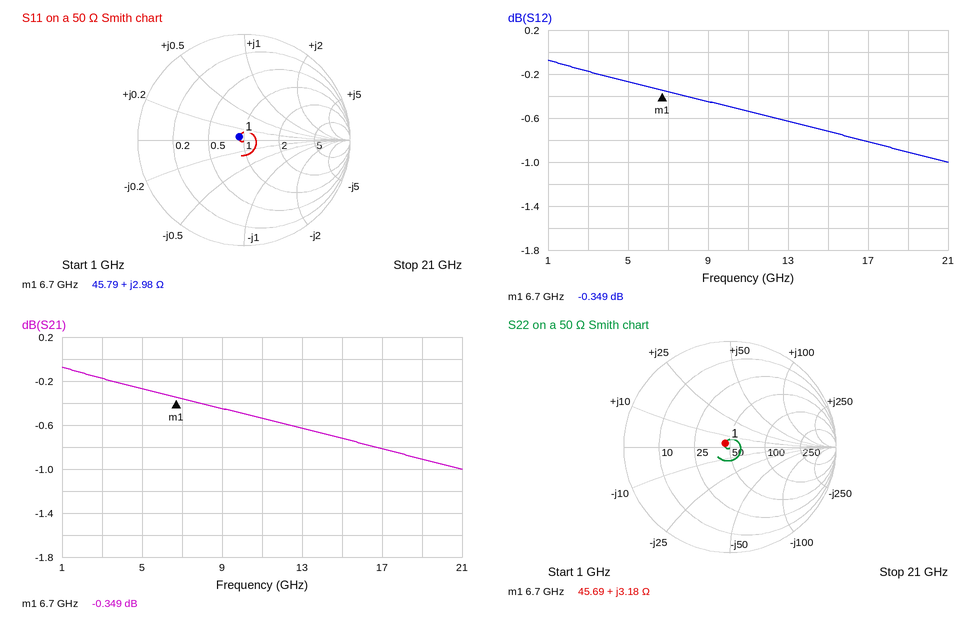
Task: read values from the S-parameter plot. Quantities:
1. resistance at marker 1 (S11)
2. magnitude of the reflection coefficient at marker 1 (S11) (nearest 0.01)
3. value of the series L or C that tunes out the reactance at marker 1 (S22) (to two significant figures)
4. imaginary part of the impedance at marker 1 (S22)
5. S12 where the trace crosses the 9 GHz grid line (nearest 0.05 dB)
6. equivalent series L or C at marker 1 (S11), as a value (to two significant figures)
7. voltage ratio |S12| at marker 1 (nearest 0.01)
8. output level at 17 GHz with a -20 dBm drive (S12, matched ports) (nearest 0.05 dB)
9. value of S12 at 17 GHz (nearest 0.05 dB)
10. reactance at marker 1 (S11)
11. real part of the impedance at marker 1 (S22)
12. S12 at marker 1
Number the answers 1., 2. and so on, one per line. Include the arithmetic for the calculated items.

1. 45.79 Ω
2. 0.05
3. C = 1/(2π × 6.7 GHz × 3.18 Ω) ≈ 7.5 pF
4. +3.18 Ω
5. -0.45 dB
6. L = 2.98 Ω/(2π × 6.7 GHz) ≈ 71 pH
7. 10^(-0.349/20) ≈ 0.96
8. -20 dBm + (-0.80 dB) = -20.80 dBm
9. -0.80 dB
10. +2.98 Ω
11. 45.69 Ω
12. -0.349 dB
